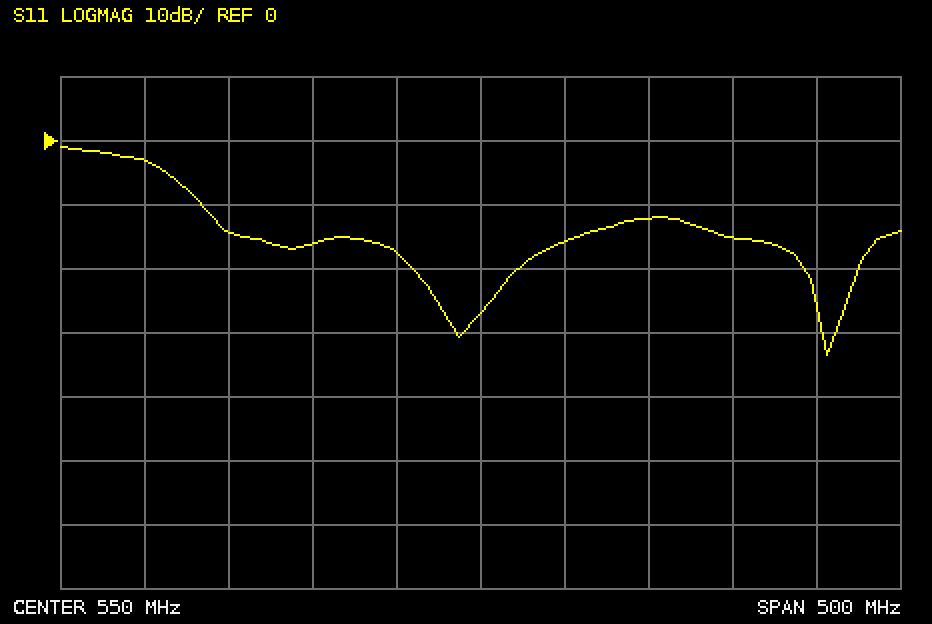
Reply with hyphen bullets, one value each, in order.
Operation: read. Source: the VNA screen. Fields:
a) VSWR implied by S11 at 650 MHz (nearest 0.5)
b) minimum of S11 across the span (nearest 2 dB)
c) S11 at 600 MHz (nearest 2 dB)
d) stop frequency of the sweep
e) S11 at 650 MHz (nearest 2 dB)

- 1.5
- -34 dB
- -16 dB
- 800 MHz
- -12 dB
